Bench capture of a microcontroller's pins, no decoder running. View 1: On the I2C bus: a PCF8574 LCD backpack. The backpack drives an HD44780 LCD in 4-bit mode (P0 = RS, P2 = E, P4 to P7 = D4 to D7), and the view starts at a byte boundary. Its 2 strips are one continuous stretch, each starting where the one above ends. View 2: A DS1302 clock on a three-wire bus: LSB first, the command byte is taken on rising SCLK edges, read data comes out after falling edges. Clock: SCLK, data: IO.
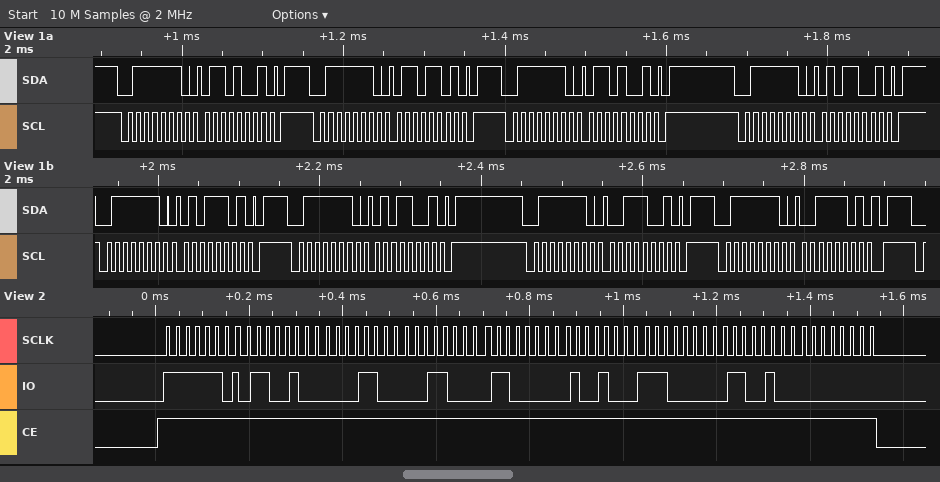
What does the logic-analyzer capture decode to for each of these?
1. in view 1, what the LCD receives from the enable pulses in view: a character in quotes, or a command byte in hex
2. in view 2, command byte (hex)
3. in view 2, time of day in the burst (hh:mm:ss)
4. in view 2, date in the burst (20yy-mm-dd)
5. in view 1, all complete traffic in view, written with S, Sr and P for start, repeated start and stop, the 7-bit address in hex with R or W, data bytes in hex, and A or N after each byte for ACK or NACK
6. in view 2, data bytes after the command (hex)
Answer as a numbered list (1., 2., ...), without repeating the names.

1. 'e'
2. 0xBF
3. 18:30:26
4. 2026-12-06
5. S 3FW A 69 A P S 3FW A 6D A P S 3FW A 69 A P S 3FW A 59 A P S 3FW A 5D A P S 3FW A 59 A P S 3FW A 39 A P S 3FW A 3D A P
6. 26 30 18 06 12 07 26 00
